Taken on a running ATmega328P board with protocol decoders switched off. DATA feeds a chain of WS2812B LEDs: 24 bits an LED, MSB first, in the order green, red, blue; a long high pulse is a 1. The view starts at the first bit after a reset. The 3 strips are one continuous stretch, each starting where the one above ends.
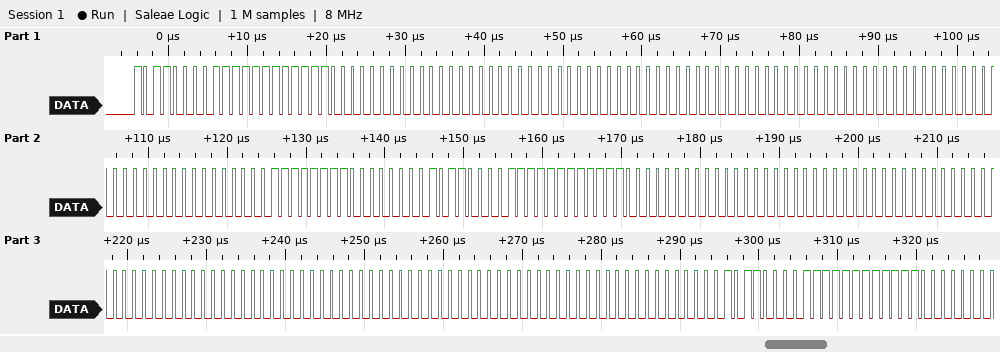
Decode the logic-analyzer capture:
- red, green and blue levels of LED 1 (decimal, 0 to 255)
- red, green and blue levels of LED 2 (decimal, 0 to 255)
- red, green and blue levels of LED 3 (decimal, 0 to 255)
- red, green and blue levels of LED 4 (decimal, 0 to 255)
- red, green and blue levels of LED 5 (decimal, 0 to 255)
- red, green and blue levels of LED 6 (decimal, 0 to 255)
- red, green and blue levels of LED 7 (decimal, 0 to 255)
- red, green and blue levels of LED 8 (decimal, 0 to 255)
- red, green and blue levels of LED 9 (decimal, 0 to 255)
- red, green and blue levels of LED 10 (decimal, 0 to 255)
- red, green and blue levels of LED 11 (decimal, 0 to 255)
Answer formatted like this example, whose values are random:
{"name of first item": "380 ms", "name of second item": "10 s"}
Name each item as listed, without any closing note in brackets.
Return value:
{"red, green and blue levels of LED 1": "255, 176, 240", "red, green and blue levels of LED 2": "0, 0, 0", "red, green and blue levels of LED 3": "0, 0, 0", "red, green and blue levels of LED 4": "0, 0, 0", "red, green and blue levels of LED 5": "255, 0, 0", "red, green and blue levels of LED 6": "255, 176, 240", "red, green and blue levels of LED 7": "0, 0, 0", "red, green and blue levels of LED 8": "0, 0, 0", "red, green and blue levels of LED 9": "0, 0, 0", "red, green and blue levels of LED 10": "0, 0, 0", "red, green and blue levels of LED 11": "255, 176, 240"}
